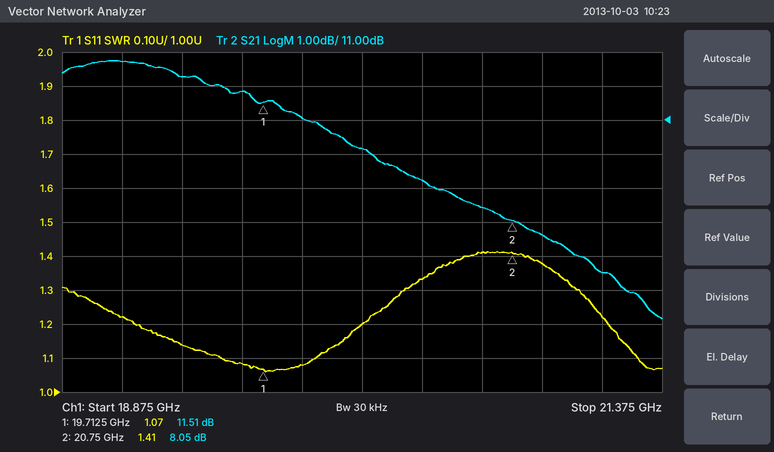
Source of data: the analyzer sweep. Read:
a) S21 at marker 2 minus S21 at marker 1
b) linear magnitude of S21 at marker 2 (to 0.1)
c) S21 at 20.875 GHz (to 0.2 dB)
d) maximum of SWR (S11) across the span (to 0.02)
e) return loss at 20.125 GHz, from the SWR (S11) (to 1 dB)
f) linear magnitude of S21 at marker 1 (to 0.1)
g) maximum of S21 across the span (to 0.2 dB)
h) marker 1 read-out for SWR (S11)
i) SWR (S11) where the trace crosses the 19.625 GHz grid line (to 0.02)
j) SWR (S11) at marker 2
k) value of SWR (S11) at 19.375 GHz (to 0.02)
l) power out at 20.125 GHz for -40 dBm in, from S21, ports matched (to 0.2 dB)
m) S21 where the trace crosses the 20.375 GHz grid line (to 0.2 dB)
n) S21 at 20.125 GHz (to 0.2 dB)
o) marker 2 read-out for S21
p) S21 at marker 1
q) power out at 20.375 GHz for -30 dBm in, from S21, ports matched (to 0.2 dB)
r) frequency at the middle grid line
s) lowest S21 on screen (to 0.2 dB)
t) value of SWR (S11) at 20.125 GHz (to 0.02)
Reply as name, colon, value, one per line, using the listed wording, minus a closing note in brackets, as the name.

S21 at marker 2 minus S21 at marker 1: -3.46 dB
linear magnitude of S21 at marker 2: 2.5
S21 at 20.875 GHz: 7.6 dB
maximum of SWR (S11) across the span: 1.42
return loss at 20.125 GHz, from the SWR (S11): 21 dB
linear magnitude of S21 at marker 1: 3.8
maximum of S21 across the span: 12.8 dB
marker 1 read-out for SWR: 1.07
SWR (S11) where the trace crosses the 19.625 GHz grid line: 1.08
SWR (S11) at marker 2: 1.41
value of SWR (S11) at 19.375 GHz: 1.14
power out at 20.125 GHz for -40 dBm in, from S21, ports matched: -29.8 dBm
S21 where the trace crosses the 20.375 GHz grid line: 9.2 dB
S21 at 20.125 GHz: 10.2 dB
marker 2 read-out for S21: 8.05 dB
S21 at marker 1: 11.51 dB
power out at 20.375 GHz for -30 dBm in, from S21, ports matched: -20.8 dBm
frequency at the middle grid line: 20.125 GHz
lowest S21 on screen: 5.2 dB
value of SWR (S11) at 20.125 GHz: 1.20
